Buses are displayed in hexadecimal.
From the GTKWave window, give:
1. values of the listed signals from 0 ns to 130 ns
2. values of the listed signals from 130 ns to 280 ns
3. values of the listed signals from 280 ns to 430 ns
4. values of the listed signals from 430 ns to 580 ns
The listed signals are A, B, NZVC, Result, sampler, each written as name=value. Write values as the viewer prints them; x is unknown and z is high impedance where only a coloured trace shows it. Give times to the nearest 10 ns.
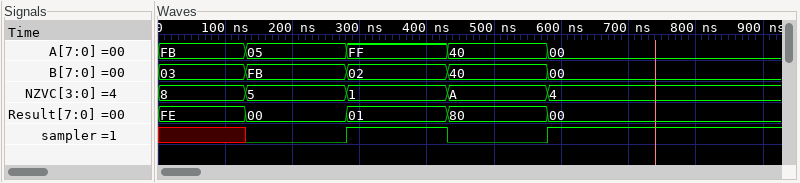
A=FB, B=03, NZVC=8, Result=FE, sampler=x
A=05, B=FB, NZVC=5, Result=00, sampler=0
A=FF, B=02, NZVC=1, Result=01, sampler=1
A=40, B=40, NZVC=A, Result=80, sampler=0
